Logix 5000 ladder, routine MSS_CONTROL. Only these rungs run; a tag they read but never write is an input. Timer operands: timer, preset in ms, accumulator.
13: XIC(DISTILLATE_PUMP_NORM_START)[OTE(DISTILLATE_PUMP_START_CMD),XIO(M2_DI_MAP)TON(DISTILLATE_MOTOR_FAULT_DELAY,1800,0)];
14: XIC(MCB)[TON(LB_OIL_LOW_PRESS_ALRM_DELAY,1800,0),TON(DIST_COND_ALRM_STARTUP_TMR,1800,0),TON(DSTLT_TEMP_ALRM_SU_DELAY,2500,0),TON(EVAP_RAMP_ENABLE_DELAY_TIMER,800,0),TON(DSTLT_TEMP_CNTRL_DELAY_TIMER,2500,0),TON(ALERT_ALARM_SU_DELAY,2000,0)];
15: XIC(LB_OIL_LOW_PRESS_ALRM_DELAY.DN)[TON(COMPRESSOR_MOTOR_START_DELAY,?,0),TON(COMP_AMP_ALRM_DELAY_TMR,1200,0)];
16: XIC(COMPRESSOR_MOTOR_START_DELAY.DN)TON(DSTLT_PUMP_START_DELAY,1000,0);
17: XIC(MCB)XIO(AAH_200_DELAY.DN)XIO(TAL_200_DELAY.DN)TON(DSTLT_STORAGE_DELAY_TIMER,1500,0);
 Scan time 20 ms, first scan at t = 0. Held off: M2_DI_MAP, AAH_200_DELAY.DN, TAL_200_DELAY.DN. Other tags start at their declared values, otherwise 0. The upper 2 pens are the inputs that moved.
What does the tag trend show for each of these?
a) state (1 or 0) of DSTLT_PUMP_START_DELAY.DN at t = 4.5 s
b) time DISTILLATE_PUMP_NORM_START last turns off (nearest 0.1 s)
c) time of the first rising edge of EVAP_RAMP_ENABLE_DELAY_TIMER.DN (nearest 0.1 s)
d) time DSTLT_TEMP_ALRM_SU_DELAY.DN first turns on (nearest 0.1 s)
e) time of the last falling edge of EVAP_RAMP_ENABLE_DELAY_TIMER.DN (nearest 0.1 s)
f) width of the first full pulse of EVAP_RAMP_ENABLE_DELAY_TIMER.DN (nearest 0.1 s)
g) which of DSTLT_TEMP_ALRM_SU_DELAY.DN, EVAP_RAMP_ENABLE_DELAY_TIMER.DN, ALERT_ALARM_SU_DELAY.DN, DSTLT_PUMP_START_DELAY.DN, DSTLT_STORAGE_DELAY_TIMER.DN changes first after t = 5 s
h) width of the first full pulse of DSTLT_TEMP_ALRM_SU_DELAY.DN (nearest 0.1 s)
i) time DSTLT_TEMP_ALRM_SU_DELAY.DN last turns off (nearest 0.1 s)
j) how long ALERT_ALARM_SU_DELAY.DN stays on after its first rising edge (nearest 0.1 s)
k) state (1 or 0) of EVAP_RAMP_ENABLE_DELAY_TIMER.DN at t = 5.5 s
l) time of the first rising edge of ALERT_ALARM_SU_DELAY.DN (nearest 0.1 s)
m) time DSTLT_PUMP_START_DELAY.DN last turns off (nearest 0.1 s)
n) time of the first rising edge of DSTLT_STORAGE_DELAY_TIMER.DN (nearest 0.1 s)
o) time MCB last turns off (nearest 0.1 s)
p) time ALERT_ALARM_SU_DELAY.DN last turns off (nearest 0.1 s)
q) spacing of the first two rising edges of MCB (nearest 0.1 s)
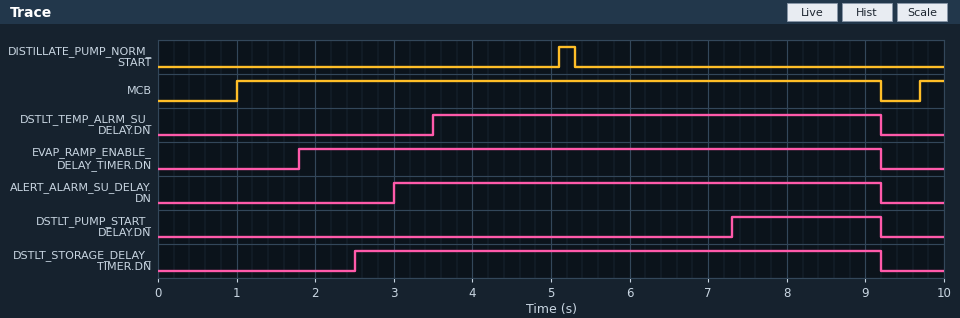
0
5.3 s
1.8 s
3.5 s
9.2 s
7.4 s
DSTLT_PUMP_START_DELAY.DN
5.7 s
9.2 s
6.2 s
1
3.0 s
9.2 s
2.5 s
9.2 s
9.2 s
8.7 s
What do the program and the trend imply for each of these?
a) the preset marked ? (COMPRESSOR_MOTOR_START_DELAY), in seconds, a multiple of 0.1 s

3.5 s
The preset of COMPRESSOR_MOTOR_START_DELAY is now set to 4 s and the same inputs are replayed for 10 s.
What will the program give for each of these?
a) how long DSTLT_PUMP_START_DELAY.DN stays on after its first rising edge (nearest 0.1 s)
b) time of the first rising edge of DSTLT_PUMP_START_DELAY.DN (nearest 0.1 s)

1.4 s
7.8 s
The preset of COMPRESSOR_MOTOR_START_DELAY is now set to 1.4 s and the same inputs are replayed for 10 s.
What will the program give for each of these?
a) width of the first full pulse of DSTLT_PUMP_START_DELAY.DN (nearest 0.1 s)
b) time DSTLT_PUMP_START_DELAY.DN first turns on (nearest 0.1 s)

4.0 s
5.2 s
